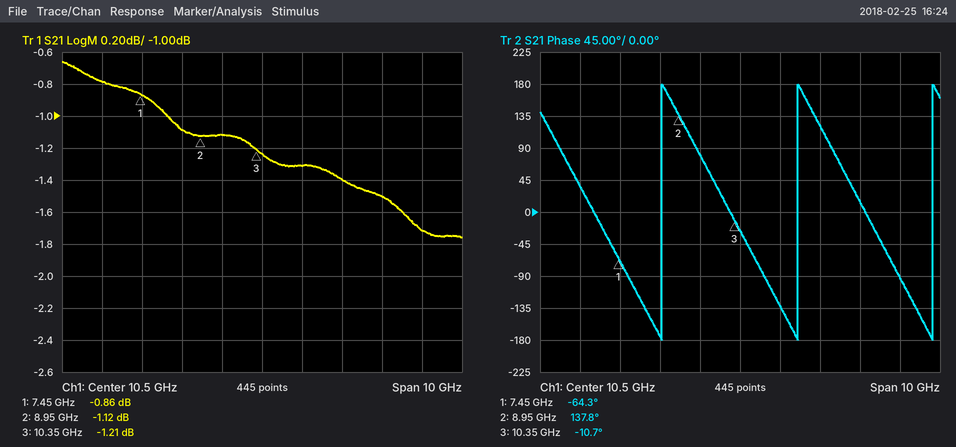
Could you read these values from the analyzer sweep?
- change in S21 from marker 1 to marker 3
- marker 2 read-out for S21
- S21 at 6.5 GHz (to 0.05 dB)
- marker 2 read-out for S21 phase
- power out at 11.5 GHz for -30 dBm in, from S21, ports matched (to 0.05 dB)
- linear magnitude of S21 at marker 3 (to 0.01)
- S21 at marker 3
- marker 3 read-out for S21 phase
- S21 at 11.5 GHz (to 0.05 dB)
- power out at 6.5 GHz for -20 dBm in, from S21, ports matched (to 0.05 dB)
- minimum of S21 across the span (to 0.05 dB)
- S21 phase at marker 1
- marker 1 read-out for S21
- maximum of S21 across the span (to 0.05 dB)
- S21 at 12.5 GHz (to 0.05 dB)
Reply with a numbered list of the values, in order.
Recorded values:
1. -0.35 dB
2. -1.12 dB
3. -0.80 dB
4. 137.8°
5. -31.30 dBm
6. 0.87
7. -1.21 dB
8. -10.7°
9. -1.30 dB
10. -20.80 dBm
11. -1.75 dB
12. -64.3°
13. -0.86 dB
14. -0.65 dB
15. -1.40 dB
